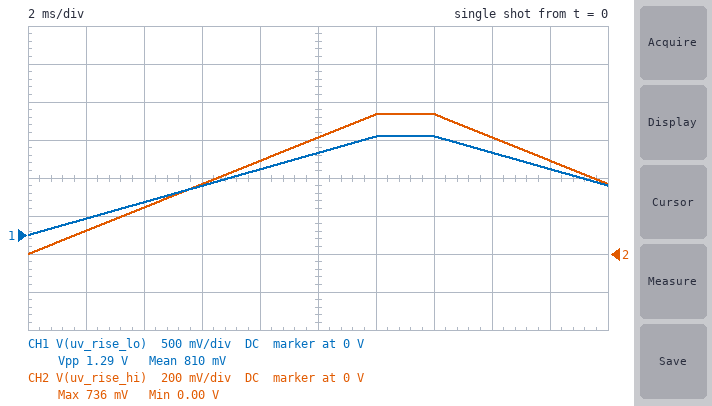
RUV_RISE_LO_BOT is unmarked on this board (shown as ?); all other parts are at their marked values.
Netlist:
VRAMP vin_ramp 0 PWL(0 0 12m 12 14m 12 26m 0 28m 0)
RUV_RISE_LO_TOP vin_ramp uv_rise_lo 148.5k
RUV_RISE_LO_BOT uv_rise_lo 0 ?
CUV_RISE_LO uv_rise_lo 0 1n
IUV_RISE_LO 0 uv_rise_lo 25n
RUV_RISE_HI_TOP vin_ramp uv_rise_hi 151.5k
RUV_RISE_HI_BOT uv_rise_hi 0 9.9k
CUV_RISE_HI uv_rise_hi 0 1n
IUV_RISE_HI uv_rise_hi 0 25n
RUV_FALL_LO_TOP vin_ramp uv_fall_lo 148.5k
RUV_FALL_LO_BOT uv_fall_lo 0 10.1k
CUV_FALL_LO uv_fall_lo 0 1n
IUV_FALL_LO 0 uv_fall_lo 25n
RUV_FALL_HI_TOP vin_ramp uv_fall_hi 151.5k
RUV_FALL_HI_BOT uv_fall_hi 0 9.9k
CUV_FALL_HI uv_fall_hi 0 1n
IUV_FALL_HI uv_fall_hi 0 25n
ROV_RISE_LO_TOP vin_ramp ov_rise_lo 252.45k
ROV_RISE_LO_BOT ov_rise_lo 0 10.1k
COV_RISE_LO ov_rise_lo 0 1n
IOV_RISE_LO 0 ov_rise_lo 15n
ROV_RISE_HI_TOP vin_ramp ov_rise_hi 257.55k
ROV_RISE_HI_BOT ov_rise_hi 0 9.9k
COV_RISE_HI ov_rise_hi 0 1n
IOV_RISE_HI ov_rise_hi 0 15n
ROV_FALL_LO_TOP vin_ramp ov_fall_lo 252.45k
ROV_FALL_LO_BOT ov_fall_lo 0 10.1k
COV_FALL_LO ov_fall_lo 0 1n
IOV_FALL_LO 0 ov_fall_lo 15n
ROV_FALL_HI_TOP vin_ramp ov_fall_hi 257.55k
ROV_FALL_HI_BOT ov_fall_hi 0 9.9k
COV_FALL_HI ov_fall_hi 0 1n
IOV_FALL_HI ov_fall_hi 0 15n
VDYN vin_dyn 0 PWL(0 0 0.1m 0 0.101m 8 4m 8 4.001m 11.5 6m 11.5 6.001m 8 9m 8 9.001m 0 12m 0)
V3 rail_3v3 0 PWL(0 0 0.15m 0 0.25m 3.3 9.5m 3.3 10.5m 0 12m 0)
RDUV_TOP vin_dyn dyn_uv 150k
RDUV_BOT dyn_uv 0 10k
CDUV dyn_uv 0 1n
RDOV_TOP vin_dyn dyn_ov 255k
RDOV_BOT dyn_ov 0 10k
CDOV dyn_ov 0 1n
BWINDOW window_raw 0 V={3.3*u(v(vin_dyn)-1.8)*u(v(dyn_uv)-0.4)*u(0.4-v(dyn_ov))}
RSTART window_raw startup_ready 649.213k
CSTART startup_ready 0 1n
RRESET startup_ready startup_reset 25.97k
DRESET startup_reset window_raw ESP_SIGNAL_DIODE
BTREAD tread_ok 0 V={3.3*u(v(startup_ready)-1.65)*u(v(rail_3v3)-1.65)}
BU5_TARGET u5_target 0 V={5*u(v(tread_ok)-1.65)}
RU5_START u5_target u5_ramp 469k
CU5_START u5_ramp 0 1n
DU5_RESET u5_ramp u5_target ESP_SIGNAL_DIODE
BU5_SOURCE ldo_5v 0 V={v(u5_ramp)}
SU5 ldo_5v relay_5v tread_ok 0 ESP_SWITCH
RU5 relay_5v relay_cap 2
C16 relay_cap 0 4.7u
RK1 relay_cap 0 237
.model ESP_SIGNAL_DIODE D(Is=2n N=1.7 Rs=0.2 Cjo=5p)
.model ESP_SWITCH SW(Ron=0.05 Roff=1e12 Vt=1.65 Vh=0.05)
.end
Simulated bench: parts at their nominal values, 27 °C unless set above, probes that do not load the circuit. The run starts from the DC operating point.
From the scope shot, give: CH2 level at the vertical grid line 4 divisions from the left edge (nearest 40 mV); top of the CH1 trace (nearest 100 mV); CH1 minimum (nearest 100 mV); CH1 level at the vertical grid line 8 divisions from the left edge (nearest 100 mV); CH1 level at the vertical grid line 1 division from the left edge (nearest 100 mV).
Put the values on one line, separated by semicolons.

480 mV; 1.3 V; 0 V; 1.1 V; 200 mV
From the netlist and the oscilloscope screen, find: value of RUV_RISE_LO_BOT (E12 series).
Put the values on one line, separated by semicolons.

18 kΩ
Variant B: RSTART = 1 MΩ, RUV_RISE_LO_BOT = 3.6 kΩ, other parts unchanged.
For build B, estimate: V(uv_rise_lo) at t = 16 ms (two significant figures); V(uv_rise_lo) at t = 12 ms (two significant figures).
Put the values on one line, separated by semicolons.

240 mV; 280 mV
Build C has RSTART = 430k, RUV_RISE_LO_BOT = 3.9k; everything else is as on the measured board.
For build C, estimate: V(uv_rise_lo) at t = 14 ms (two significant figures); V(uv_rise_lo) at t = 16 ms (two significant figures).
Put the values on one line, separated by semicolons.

310 mV; 260 mV
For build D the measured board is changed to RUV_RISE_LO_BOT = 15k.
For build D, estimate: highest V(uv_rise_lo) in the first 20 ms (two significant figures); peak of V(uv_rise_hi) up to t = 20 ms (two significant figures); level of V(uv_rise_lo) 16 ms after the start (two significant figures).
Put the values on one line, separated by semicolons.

1.1 V; 740 mV; 920 mV
